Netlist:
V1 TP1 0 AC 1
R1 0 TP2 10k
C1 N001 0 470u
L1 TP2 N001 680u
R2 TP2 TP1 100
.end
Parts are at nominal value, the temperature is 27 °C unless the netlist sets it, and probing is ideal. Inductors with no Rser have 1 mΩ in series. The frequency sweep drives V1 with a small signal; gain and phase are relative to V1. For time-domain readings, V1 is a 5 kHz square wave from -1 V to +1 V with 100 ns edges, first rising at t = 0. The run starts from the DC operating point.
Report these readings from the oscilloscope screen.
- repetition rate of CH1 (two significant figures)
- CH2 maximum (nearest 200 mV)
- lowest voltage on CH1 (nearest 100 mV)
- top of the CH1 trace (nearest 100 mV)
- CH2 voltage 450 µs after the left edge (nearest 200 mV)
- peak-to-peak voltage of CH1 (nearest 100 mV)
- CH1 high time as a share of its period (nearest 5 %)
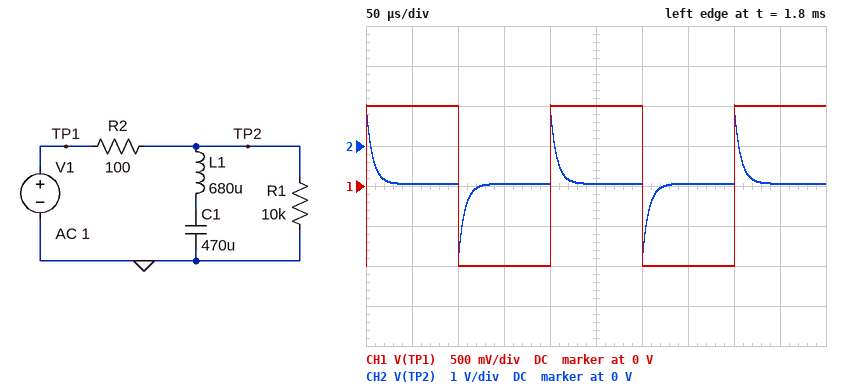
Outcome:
5.0 kHz
1.0 V
-1.0 V
1.0 V
-1.0 V
2.0 V
50 %
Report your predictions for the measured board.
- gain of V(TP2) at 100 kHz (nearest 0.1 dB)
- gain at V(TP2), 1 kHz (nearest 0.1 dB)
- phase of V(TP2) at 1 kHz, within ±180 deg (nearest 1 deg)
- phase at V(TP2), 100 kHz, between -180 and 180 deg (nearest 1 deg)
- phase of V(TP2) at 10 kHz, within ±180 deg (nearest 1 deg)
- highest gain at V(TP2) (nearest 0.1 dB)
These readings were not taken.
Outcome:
-0.3 dB
-28.1 dB
88 deg
13 deg
67 deg
-0.1 dB
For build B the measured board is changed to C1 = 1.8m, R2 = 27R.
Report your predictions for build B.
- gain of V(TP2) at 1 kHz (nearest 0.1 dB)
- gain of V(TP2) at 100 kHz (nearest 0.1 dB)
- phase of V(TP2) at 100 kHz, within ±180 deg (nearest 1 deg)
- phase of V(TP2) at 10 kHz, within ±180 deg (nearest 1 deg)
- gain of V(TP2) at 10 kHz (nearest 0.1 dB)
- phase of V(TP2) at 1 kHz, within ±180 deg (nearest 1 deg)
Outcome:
-16.3 dB
0 dB
4 deg
32 deg
-1.5 dB
81 deg
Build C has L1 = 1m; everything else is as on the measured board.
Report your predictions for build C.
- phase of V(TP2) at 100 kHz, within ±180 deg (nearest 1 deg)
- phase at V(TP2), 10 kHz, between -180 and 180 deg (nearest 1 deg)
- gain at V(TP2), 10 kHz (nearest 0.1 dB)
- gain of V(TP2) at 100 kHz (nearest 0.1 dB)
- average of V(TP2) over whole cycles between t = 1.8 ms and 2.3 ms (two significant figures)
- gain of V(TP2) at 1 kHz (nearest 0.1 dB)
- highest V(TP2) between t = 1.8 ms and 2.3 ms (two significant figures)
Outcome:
9 deg
58 deg
-5.5 dB
-0.2 dB
-910 mV
-24.5 dB
1.0 V
